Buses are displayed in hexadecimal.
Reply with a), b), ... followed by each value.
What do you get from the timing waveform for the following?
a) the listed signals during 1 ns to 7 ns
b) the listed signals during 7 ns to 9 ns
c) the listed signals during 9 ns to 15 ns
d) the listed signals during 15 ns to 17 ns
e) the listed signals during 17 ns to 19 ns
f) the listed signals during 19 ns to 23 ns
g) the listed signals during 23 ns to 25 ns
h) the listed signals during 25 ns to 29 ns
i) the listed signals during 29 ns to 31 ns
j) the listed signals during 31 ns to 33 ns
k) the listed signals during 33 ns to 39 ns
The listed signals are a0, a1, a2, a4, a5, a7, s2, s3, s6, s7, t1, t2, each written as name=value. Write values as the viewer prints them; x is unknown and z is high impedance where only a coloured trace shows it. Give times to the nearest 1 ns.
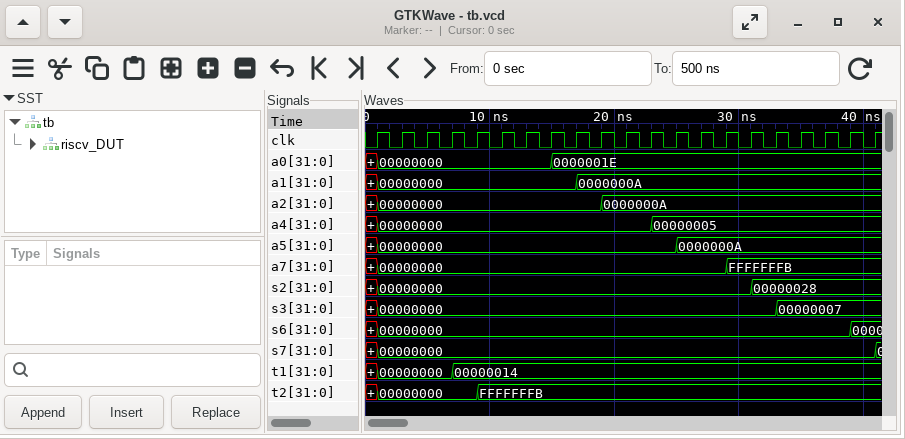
a) a0=00000000, a1=00000000, a2=00000000, a4=00000000, a5=00000000, a7=00000000, s2=00000000, s3=00000000, s6=00000000, s7=00000000, t1=00000000, t2=00000000
b) a0=00000000, a1=00000000, a2=00000000, a4=00000000, a5=00000000, a7=00000000, s2=00000000, s3=00000000, s6=00000000, s7=00000000, t1=00000014, t2=00000000
c) a0=00000000, a1=00000000, a2=00000000, a4=00000000, a5=00000000, a7=00000000, s2=00000000, s3=00000000, s6=00000000, s7=00000000, t1=00000014, t2=FFFFFFFB
d) a0=0000001E, a1=00000000, a2=00000000, a4=00000000, a5=00000000, a7=00000000, s2=00000000, s3=00000000, s6=00000000, s7=00000000, t1=00000014, t2=FFFFFFFB
e) a0=0000001E, a1=0000000A, a2=00000000, a4=00000000, a5=00000000, a7=00000000, s2=00000000, s3=00000000, s6=00000000, s7=00000000, t1=00000014, t2=FFFFFFFB
f) a0=0000001E, a1=0000000A, a2=0000000A, a4=00000000, a5=00000000, a7=00000000, s2=00000000, s3=00000000, s6=00000000, s7=00000000, t1=00000014, t2=FFFFFFFB
g) a0=0000001E, a1=0000000A, a2=0000000A, a4=00000005, a5=00000000, a7=00000000, s2=00000000, s3=00000000, s6=00000000, s7=00000000, t1=00000014, t2=FFFFFFFB
h) a0=0000001E, a1=0000000A, a2=0000000A, a4=00000005, a5=0000000A, a7=00000000, s2=00000000, s3=00000000, s6=00000000, s7=00000000, t1=00000014, t2=FFFFFFFB
i) a0=0000001E, a1=0000000A, a2=0000000A, a4=00000005, a5=0000000A, a7=FFFFFFFB, s2=00000000, s3=00000000, s6=00000000, s7=00000000, t1=00000014, t2=FFFFFFFB
j) a0=0000001E, a1=0000000A, a2=0000000A, a4=00000005, a5=0000000A, a7=FFFFFFFB, s2=00000028, s3=00000000, s6=00000000, s7=00000000, t1=00000014, t2=FFFFFFFB
k) a0=0000001E, a1=0000000A, a2=0000000A, a4=00000005, a5=0000000A, a7=FFFFFFFB, s2=00000028, s3=00000007, s6=00000000, s7=00000000, t1=00000014, t2=FFFFFFFB
